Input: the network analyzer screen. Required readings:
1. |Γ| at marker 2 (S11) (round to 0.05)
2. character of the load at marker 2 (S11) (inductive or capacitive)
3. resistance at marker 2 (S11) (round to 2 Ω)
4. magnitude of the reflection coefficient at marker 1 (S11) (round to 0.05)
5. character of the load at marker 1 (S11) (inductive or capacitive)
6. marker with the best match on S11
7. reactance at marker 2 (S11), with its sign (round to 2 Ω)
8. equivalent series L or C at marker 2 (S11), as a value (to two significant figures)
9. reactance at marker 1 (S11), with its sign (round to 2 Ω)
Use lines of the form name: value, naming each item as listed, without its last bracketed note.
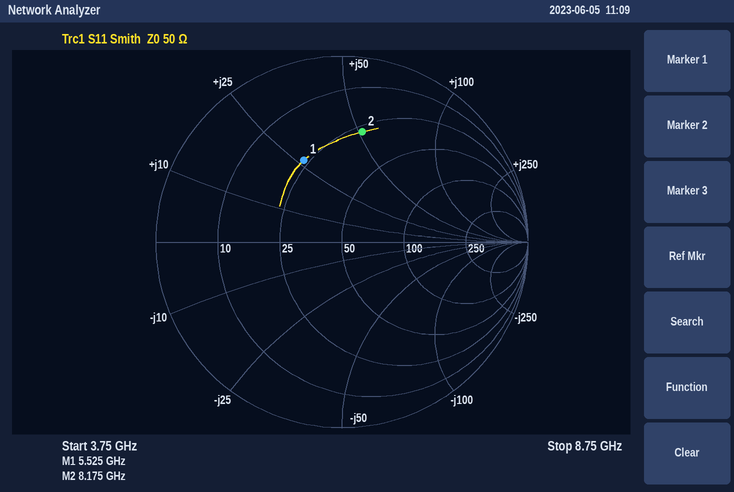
|Γ| at marker 2 (S11): 0.60
character of the load at marker 2 (S11): inductive
resistance at marker 2 (S11): 28 Ω
magnitude of the reflection coefficient at marker 1 (S11): 0.50
character of the load at marker 1 (S11): inductive
marker with the best match on S11: marker 1
reactance at marker 2 (S11), with its sign: +52 Ω
equivalent series L or C at marker 2 (S11), as a value: 1.0 nH
reactance at marker 1 (S11), with its sign: +26 Ω
